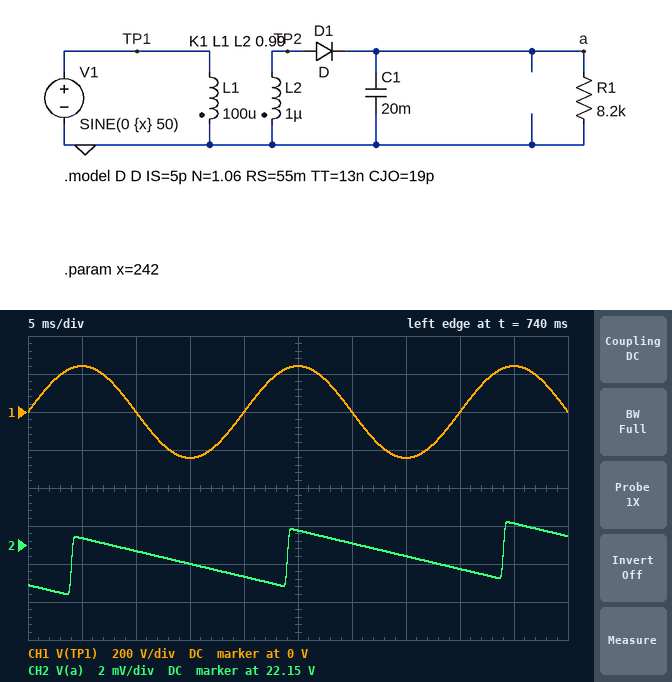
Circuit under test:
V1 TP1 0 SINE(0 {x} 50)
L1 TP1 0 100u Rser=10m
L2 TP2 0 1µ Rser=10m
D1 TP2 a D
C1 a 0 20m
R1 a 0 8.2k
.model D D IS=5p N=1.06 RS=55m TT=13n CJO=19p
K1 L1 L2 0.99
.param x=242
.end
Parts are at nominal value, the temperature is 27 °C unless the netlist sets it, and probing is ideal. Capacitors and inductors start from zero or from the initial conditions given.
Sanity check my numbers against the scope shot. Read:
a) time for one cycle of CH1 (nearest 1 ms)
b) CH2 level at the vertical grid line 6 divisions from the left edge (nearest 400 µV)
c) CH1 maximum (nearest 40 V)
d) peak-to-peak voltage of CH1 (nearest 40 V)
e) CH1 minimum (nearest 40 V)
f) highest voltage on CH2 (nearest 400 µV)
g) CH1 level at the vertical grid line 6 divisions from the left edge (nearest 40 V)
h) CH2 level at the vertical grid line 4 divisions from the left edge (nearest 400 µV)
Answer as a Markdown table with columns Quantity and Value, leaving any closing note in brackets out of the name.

| Quantity | Value |
|---|---|
| time for one cycle of CH1 | 20 ms |
| CH2 level at the vertical grid line 6 divisions from the left edge | 22.1480 V |
| CH1 maximum | 240 V |
| peak-to-peak voltage of CH1 | 480 V |
| CH1 minimum | -240 V |
| highest voltage on CH2 | 22.1492 V |
| CH1 level at the vertical grid line 6 divisions from the left edge | 0 V |
| CH2 level at the vertical grid line 4 divisions from the left edge | 22.1464 V |
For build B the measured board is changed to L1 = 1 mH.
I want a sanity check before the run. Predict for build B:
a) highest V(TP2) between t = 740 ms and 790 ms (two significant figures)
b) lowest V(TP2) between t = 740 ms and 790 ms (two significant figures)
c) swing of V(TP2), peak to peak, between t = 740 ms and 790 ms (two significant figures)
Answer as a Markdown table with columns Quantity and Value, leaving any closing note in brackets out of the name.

| Quantity | Value |
|---|---|
| highest V(TP2) between t = 740 ms and 790 ms | 7.6 V |
| lowest V(TP2) between t = 740 ms and 790 ms | -7.6 V |
| swing of V(TP2), peak to peak, between t = 740 ms and 790 ms | 15 V |
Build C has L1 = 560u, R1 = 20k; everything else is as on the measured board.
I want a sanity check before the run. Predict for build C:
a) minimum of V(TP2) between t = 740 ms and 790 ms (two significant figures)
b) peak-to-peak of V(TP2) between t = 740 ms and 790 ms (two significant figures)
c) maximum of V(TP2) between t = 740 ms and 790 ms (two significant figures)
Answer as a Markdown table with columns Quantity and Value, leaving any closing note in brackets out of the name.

| Quantity | Value |
|---|---|
| minimum of V(TP2) between t = 740 ms and 790 ms | -10 V |
| peak-to-peak of V(TP2) between t = 740 ms and 790 ms | 20 V |
| maximum of V(TP2) between t = 740 ms and 790 ms | 10 V |
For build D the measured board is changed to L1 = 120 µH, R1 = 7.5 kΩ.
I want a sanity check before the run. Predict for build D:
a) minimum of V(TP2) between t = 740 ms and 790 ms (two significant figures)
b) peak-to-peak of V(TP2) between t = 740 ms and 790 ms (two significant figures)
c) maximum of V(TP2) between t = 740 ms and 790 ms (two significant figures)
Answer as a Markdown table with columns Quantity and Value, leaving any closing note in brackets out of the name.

| Quantity | Value |
|---|---|
| minimum of V(TP2) between t = 740 ms and 790 ms | -21 V |
| peak-to-peak of V(TP2) between t = 740 ms and 790 ms | 42 V |
| maximum of V(TP2) between t = 740 ms and 790 ms | 21 V |
